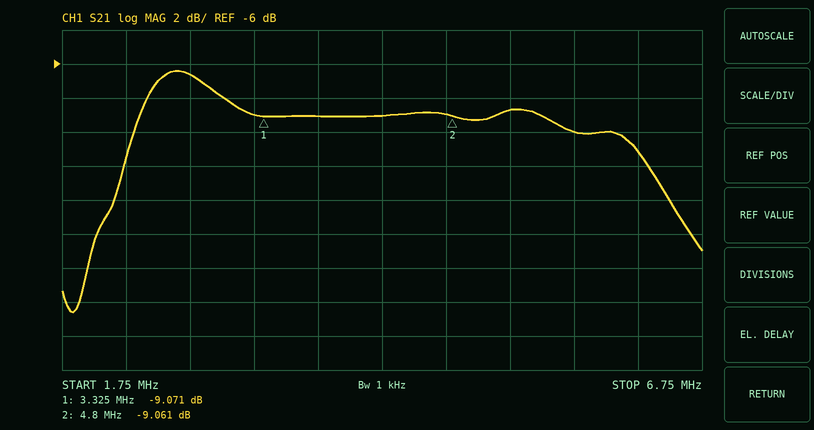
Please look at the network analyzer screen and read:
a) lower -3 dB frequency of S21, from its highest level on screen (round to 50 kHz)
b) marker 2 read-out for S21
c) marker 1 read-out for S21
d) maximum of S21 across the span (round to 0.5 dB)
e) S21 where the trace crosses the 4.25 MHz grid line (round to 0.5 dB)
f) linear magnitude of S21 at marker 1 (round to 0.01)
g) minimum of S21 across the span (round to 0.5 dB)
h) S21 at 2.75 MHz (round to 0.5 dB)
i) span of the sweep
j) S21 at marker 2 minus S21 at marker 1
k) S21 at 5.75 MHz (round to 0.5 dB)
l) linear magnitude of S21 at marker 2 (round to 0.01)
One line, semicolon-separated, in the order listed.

2.35 MHz; -9.061 dB; -9.071 dB; -6.5 dB; -9.0 dB; 0.35; -20.5 dB; -6.5 dB; 5 MHz; 0.010 dB; -10.0 dB; 0.35
